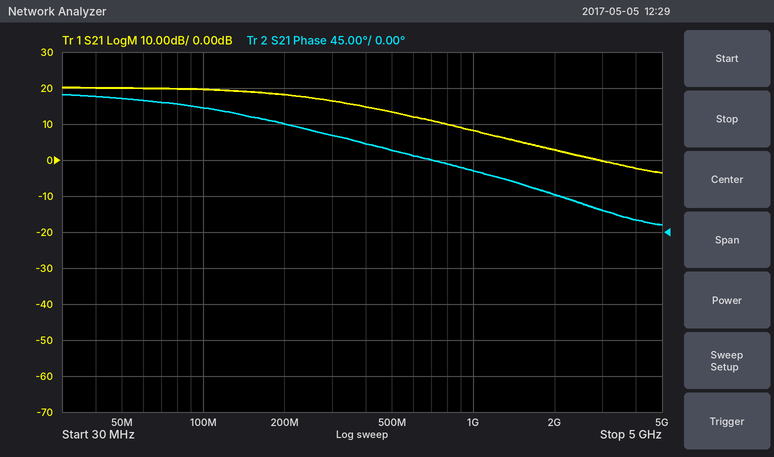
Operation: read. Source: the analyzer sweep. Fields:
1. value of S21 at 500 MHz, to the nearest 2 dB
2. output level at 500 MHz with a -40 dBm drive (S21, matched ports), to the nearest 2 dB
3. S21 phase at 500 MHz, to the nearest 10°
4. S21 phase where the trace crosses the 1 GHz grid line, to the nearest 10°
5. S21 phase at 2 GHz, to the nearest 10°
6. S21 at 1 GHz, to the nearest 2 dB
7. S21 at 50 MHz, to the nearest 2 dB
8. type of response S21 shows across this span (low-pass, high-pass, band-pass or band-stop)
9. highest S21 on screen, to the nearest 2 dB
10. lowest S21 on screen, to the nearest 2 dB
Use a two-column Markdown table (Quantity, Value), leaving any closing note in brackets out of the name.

| Quantity | Value |
|---|---|
| value of S21 at 500 MHz, to the nearest 2 dB | 14 dB |
| output level at 500 MHz with a -40 dBm drive (S21, matched ports), to the nearest 2 dB | -26 dBm |
| S21 phase at 500 MHz, to the nearest 10° | 100° |
| S21 phase where the trace crosses the 1 GHz grid line, to the nearest 10° | 80° |
| S21 phase at 2 GHz, to the nearest 10° | 50° |
| S21 at 1 GHz, to the nearest 2 dB | 8 dB |
| S21 at 50 MHz, to the nearest 2 dB | 20 dB |
| type of response S21 shows across this span | low-pass |
| highest S21 on screen, to the nearest 2 dB | 20 dB |
| lowest S21 on screen, to the nearest 2 dB | -4 dB |
